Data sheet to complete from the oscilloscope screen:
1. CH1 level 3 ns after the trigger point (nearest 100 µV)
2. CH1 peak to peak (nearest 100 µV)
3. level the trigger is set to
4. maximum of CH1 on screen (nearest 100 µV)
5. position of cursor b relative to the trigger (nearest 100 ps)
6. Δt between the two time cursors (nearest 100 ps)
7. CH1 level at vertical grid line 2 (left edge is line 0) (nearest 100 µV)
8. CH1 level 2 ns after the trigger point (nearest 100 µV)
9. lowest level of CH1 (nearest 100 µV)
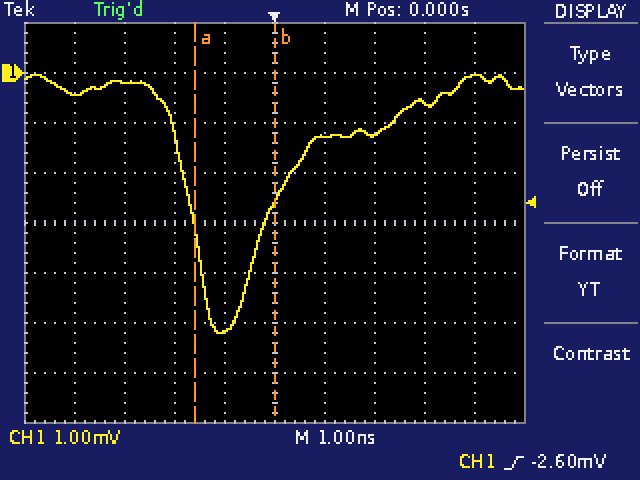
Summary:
-600 µV
5.2 mV
-2.60 mV
0.0 mV
0.0 ns
1.6 ns
-200 µV
-1.2 mV
-5.2 mV
